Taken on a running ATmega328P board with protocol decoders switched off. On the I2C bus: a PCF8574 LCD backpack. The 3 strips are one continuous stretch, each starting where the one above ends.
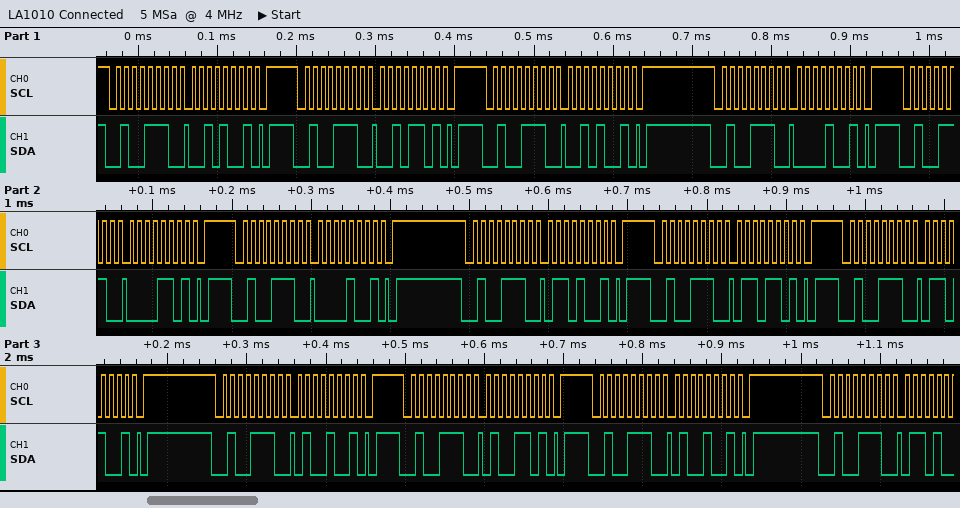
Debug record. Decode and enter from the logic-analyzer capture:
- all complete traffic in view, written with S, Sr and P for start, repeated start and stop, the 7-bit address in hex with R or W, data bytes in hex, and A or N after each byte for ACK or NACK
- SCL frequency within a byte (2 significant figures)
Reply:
S 27W A 29 A P S 27W A 2D A P S 27W A 29 A P S 27W A 09 A P S 27W A 0D A P S 27W A 09 A P S 27W A 69 A P S 27W A 6D A P S 27W A 69 A P S 27W A 49 A P S 27W A 4D A P S 27W A 49 A P S 27W A
100 kHz
